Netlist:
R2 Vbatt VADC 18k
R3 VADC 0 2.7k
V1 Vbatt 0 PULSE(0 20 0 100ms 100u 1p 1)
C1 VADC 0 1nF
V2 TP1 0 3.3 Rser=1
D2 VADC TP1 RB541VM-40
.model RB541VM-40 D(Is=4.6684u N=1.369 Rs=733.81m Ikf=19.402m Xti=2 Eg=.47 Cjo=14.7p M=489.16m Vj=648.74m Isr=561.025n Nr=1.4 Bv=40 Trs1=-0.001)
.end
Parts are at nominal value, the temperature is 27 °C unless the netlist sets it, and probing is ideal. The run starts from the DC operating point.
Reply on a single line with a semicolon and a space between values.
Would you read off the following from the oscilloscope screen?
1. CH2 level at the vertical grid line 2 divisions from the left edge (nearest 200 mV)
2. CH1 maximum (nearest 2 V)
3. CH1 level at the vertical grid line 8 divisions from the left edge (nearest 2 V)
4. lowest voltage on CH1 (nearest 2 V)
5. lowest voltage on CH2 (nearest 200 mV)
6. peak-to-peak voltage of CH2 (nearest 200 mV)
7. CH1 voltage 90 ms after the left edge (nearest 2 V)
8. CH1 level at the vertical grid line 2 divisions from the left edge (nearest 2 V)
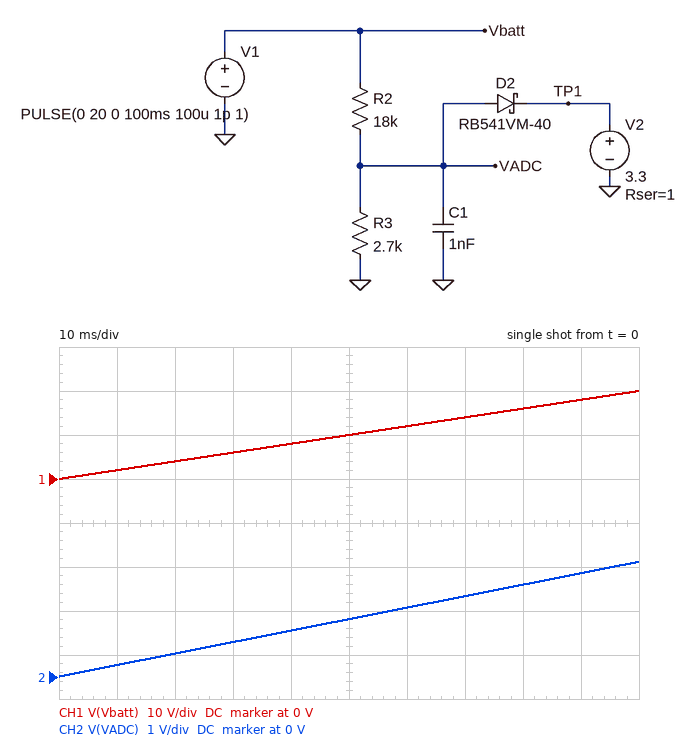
600 mV; 20 V; 16 V; 0 V; 0 V; 2.6 V; 18 V; 4 V
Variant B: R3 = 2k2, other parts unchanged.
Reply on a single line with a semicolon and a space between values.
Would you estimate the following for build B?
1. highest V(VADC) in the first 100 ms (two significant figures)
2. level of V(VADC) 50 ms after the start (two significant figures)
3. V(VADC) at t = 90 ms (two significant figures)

2.2 V; 1.1 V; 2.0 V
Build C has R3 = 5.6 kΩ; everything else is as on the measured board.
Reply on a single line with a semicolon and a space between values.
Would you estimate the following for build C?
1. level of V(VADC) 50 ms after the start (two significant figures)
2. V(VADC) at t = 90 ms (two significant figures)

2.4 V; 3.4 V
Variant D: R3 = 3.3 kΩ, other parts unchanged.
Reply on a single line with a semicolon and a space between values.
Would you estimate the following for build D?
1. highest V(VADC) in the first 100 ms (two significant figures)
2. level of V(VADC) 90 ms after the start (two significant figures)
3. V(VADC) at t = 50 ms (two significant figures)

3.1 V; 2.8 V; 1.6 V
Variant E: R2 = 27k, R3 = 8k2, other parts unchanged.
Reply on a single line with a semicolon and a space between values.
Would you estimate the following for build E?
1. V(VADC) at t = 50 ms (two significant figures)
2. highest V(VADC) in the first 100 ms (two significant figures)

2.4 V; 3.4 V
